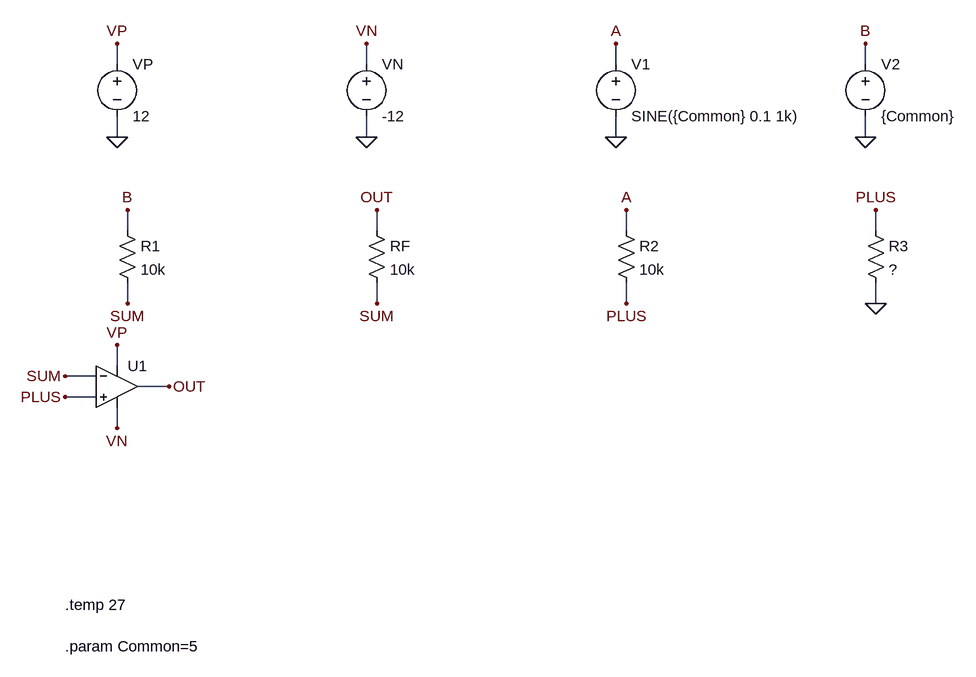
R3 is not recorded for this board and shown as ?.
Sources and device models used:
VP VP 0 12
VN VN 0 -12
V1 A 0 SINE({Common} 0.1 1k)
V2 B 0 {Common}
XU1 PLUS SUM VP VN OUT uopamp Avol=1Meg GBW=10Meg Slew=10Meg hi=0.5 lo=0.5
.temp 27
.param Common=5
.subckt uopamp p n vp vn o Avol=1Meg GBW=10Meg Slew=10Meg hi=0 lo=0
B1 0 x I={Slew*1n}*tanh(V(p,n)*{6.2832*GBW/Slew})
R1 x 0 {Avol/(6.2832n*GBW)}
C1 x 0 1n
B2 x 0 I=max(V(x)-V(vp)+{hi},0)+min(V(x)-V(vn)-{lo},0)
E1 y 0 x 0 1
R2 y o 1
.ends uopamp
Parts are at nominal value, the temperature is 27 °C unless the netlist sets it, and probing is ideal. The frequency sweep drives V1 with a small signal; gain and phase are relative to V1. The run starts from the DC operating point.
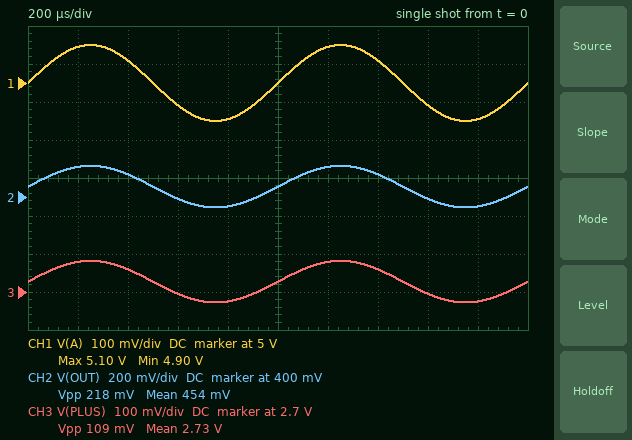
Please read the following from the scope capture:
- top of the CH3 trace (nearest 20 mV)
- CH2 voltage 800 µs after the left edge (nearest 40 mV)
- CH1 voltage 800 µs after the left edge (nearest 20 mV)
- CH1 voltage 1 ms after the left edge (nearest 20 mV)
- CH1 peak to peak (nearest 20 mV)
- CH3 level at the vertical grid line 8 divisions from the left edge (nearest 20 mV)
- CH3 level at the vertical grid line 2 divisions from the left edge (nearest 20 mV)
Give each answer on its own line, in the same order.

2.78 V
360 mV
4.90 V
5.00 V
200 mV
2.70 V
2.76 V
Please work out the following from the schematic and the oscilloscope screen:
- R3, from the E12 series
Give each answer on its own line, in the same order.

12 kΩ
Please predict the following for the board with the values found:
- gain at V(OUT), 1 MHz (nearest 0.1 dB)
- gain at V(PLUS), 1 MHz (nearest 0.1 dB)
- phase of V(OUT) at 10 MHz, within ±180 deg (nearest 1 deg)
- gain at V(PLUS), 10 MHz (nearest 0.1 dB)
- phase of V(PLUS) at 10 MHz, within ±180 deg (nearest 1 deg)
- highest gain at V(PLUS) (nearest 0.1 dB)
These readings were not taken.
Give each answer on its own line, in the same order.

0.6 dB
-5.3 dB
-63 deg
-5.3 dB
0 deg
-5.3 dB
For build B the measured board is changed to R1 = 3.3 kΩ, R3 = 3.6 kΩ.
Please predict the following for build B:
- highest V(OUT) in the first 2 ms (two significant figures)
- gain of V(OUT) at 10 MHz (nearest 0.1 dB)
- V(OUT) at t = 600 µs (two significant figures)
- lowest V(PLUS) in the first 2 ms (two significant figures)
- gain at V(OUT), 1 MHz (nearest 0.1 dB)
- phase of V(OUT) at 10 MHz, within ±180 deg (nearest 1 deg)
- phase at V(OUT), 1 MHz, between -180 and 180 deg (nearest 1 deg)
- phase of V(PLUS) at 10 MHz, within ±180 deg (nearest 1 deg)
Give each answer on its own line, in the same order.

-9.7 V
-11.8 dB
-9.9 V
1.3 V
-0.1 dB
-76 deg
-22 deg
0 deg
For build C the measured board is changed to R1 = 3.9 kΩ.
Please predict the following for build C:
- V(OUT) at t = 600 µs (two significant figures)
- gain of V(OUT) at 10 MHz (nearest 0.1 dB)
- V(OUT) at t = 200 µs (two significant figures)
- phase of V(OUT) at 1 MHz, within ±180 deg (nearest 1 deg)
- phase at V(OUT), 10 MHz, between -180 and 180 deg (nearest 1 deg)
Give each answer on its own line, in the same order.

-3.2 V
-5.6 dB
-2.9 V
-20 deg
-74 deg
